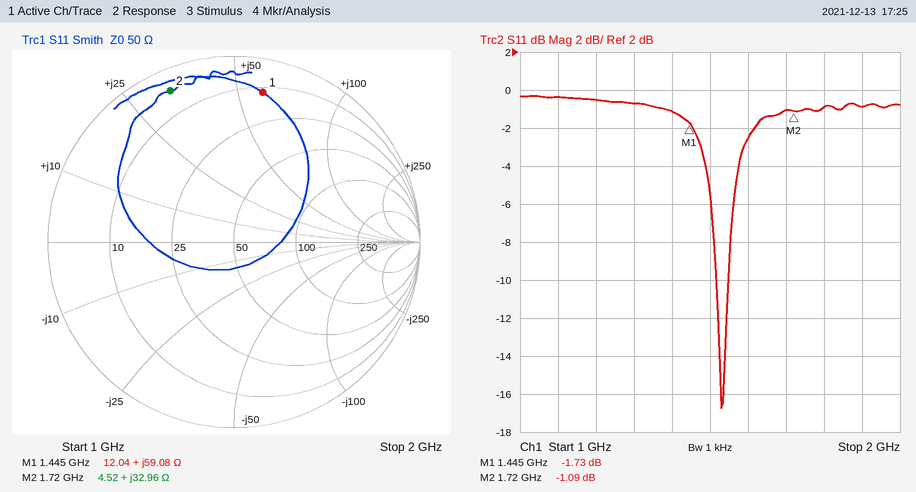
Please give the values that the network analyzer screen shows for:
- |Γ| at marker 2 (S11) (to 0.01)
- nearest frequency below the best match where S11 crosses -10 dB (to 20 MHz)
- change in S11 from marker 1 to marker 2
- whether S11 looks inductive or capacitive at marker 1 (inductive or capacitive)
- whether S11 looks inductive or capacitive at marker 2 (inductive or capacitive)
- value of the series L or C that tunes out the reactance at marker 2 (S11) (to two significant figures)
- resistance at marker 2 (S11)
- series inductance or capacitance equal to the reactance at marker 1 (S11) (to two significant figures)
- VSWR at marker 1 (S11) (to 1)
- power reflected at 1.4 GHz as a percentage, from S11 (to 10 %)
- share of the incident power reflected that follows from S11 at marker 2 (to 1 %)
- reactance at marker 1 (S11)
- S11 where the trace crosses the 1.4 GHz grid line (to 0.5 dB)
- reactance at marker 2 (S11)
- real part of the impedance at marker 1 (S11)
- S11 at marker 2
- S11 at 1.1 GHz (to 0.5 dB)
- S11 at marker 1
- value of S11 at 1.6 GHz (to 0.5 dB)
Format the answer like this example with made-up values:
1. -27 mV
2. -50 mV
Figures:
1. 0.88
2. 1.52 GHz
3. 0.64 dB
4. inductive
5. inductive
6. 2.8 pF
7. 4.52 Ω
8. 6.5 nH
9. 10
10. 80 %
11. 78 %
12. +59.08 Ω
13. -1.0 dB
14. +32.96 Ω
15. 12.04 Ω
16. -1.09 dB
17. -0.5 dB
18. -1.73 dB
19. -2.5 dB
